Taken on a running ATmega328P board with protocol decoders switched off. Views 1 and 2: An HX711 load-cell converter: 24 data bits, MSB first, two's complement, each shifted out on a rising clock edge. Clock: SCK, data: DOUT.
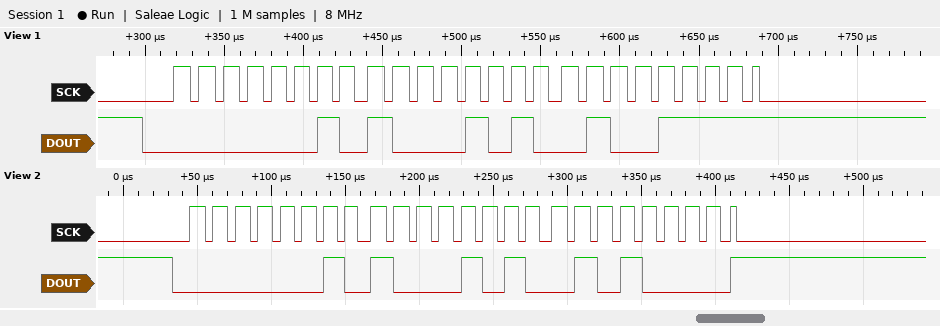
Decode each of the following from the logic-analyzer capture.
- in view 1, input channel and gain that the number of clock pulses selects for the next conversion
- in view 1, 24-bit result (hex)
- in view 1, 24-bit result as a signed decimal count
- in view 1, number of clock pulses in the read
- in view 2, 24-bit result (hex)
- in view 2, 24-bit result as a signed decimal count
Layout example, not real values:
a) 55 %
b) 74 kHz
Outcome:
a) channel A, gain 128
b) 0x028A4F
c) 166479
d) 25
e) 0x028A50
f) 166480
